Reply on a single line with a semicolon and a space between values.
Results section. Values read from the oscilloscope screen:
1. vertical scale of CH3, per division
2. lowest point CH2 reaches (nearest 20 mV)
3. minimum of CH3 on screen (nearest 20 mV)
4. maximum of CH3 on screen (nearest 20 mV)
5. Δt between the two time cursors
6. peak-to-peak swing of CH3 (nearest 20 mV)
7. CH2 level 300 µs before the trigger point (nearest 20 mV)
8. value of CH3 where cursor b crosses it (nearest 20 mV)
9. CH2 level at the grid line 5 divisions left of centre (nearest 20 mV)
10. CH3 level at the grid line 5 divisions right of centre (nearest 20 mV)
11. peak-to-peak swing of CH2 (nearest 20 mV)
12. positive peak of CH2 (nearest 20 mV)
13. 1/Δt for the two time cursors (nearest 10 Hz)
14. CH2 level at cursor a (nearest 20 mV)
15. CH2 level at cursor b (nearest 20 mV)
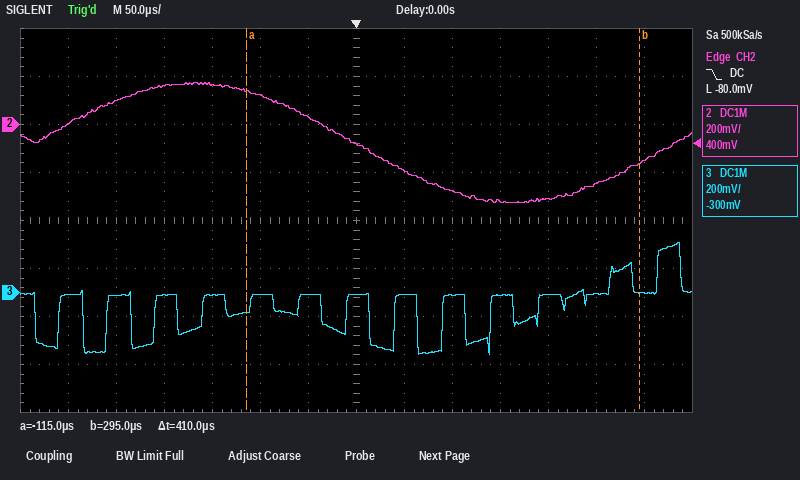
200 mV; -320 mV; -260 mV; 200 mV; 410 µs; 460 mV; 0 mV; 0 mV; 100 mV; 0 mV; 500 mV; 180 mV; 2.44 kHz; 140 mV; -160 mV
